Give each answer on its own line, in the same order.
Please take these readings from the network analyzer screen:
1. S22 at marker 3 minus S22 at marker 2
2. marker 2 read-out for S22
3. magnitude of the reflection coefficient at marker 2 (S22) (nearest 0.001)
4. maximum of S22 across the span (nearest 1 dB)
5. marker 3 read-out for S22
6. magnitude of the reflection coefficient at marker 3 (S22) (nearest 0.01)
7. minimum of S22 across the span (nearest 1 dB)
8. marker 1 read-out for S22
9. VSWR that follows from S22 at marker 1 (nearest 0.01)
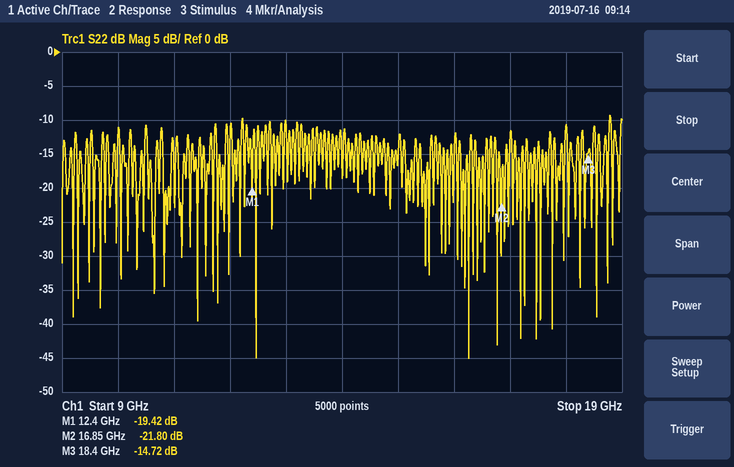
7.08 dB
-21.80 dB
0.081
-9 dB
-14.72 dB
0.18
-45 dB
-19.42 dB
1.24
